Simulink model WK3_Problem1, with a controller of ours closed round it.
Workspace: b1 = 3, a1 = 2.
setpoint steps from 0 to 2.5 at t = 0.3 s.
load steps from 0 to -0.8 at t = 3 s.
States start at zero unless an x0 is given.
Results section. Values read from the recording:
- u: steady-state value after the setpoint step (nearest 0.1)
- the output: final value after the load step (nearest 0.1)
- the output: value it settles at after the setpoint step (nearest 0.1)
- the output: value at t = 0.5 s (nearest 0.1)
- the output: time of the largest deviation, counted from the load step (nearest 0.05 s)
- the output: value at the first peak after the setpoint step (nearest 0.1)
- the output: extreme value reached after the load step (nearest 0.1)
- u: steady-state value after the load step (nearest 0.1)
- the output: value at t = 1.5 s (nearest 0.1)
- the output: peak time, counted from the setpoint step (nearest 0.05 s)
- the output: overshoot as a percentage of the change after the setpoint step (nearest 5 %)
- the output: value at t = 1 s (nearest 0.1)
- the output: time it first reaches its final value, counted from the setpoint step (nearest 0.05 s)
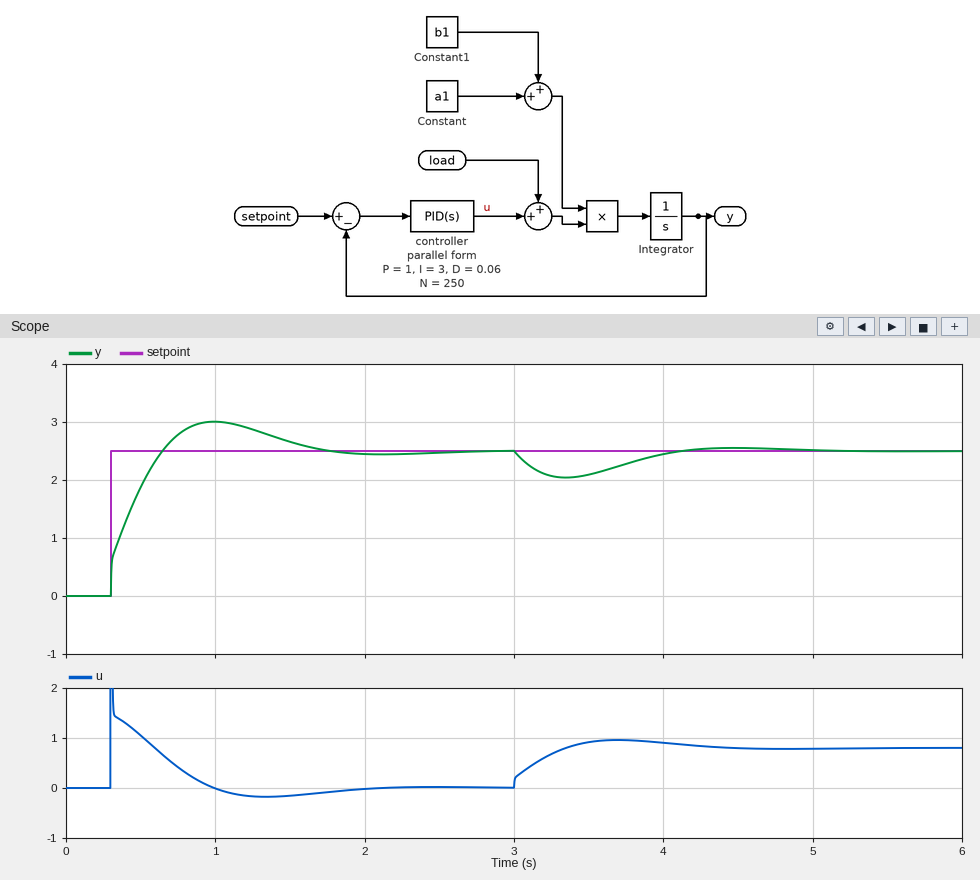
0.0
2.5
2.5
1.9
0.35 s
3.0
2.0
0.8
2.7
0.70 s
20 %
3.0
0.35 s
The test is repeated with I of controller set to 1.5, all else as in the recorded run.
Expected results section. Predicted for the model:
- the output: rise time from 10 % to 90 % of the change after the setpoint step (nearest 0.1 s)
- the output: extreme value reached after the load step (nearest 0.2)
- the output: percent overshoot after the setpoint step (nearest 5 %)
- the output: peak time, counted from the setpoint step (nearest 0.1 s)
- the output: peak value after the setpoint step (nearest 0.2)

0.3 s
2.0
15 %
0.9 s
2.8
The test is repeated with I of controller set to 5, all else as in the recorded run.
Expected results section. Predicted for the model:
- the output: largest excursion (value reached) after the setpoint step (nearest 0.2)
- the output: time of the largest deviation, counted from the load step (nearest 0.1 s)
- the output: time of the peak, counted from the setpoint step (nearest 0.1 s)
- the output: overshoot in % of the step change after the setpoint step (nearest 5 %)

3.2
0.3 s
0.6 s
25 %
